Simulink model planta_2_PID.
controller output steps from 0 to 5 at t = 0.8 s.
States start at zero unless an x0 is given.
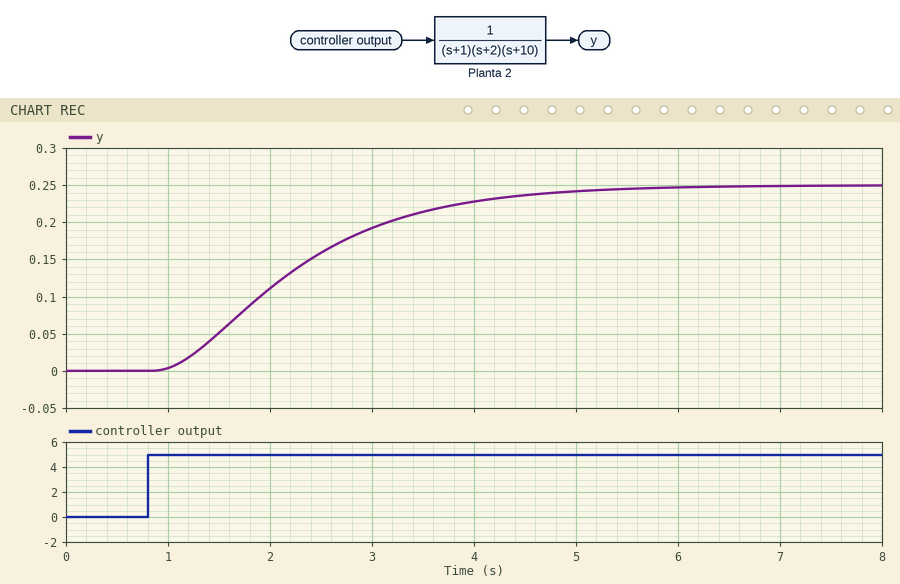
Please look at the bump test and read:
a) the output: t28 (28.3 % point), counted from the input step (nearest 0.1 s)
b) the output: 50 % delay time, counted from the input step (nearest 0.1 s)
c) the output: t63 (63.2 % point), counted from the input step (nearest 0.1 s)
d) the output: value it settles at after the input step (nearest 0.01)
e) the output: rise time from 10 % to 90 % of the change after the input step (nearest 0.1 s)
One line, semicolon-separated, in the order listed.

0.9 s; 1.3 s; 1.7 s; 0.25; 2.6 s
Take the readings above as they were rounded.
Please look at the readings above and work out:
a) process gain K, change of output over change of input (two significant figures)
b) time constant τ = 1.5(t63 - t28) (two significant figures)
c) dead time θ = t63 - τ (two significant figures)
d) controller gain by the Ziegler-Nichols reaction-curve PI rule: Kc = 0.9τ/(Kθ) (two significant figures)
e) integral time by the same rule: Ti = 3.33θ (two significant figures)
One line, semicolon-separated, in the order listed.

0.050; 1.2 s; 0.50 s; 43; 1.7 s
